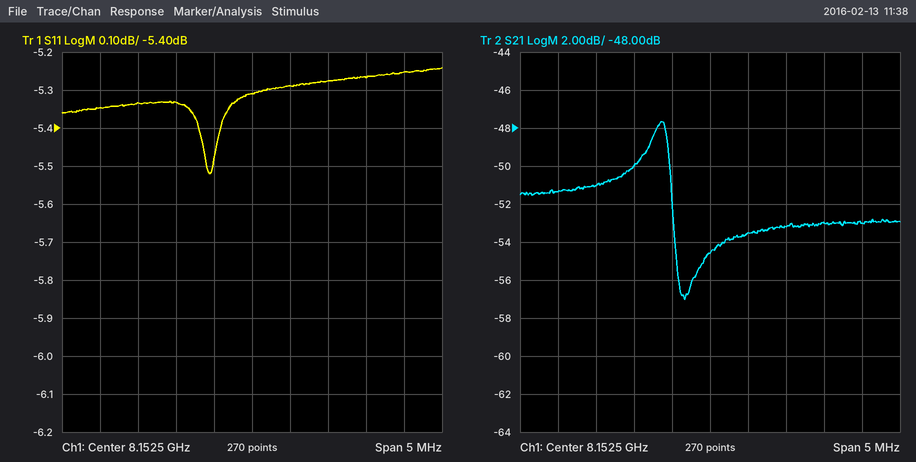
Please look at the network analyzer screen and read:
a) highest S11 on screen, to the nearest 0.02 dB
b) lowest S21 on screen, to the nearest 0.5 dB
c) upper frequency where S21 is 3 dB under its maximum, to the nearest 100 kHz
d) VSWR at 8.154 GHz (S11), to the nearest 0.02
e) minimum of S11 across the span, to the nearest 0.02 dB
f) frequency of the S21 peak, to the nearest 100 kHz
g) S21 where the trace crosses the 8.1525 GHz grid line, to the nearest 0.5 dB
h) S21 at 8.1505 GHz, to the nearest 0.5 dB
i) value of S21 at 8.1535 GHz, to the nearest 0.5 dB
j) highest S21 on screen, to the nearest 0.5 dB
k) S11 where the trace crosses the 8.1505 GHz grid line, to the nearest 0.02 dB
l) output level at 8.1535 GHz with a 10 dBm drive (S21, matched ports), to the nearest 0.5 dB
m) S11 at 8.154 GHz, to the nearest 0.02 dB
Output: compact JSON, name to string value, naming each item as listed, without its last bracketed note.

{"highest S11 on screen, to the nearest 0.02 dB": "-5.24 dB", "lowest S21 on screen, to the nearest 0.5 dB": "-57.0 dB", "upper frequency where S21 is 3 dB under its maximum, to the nearest 100 kHz": "8.1520 GHz", "VSWR at 8.154 GHz (S11), to the nearest 0.02": "3.40", "minimum of S11 across the span, to the nearest 0.02 dB": "-5.52 dB", "frequency of the S21 peak, to the nearest 100 kHz": "8.1519 GHz", "S21 where the trace crosses the 8.1525 GHz grid line, to the nearest 0.5 dB": "-54.5 dB", "S21 at 8.1505 GHz, to the nearest 0.5 dB": "-51.5 dB", "value of S21 at 8.1535 GHz, to the nearest 0.5 dB": "-53.0 dB", "highest S21 on screen, to the nearest 0.5 dB": "-47.5 dB", "S11 where the trace crosses the 8.1505 GHz grid line, to the nearest 0.02 dB": "-5.34 dB", "output level at 8.1535 GHz with a 10 dBm drive (S21, matched ports), to the nearest 0.5 dB": "-43.0 dBm", "S11 at 8.154 GHz, to the nearest 0.02 dB": "-5.26 dB"}
